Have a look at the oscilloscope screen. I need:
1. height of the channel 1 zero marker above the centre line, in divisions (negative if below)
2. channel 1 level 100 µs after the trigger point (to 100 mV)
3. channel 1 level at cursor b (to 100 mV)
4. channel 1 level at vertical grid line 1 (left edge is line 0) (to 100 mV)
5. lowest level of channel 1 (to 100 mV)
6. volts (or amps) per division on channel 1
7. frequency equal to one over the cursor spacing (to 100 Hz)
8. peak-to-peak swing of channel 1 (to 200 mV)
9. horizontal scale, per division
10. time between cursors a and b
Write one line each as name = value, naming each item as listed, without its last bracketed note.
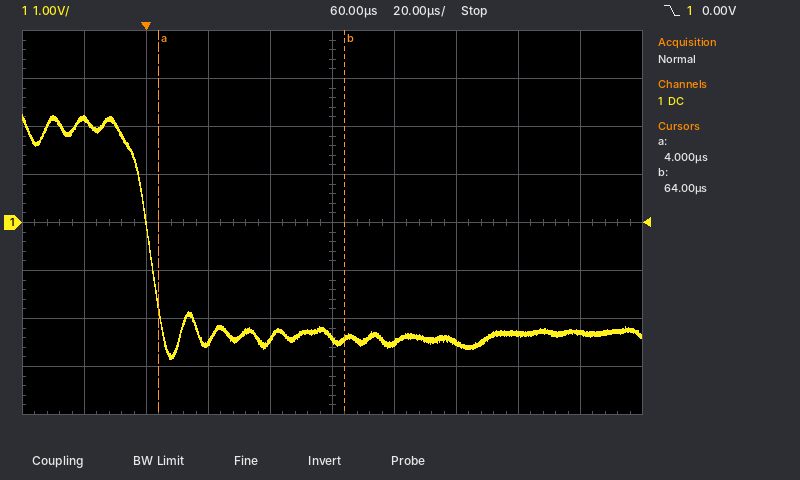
height of the channel 1 zero marker above the centre line, in divisions = 0.0 div
channel 1 level 100 µs after the trigger point = -2.5 V
channel 1 level at cursor b = -2.4 V
channel 1 level at vertical grid line 1 (left edge is line 0) = 2.2 V
lowest level of channel 1 = -2.8 V
volts (or amps) per division on channel 1 = 1 V
frequency equal to one over the cursor spacing = 16.7 kHz
peak-to-peak swing of channel 1 = 5.0 V
horizontal scale, per division = 20 µs
time between cursors a and b = 60 µs
